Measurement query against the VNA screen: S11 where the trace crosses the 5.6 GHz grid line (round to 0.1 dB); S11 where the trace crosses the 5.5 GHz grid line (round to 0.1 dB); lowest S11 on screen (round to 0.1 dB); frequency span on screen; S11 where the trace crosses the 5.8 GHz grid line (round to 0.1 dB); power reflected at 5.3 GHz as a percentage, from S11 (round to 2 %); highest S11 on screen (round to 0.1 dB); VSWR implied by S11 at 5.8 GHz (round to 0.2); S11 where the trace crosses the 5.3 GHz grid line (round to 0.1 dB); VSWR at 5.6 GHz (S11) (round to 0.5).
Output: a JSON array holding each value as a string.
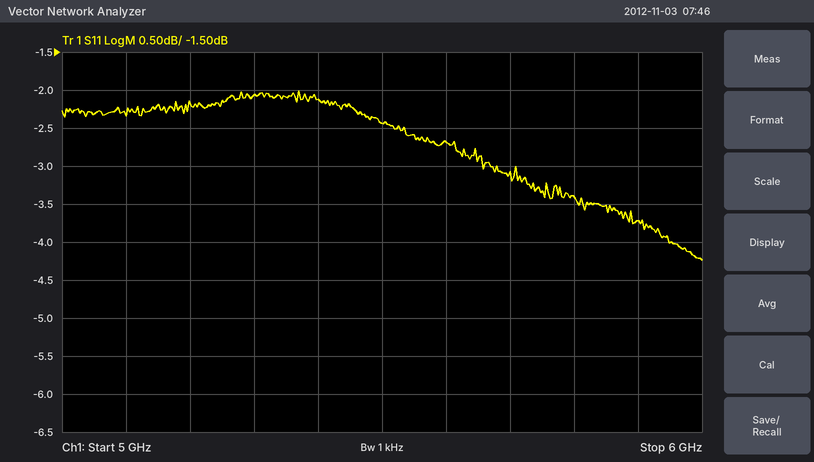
["-2.7 dB", "-2.4 dB", "-4.2 dB", "1 GHz", "-3.4 dB", "62 %", "-2.0 dB", "5.2", "-2.1 dB", "6.5"]
